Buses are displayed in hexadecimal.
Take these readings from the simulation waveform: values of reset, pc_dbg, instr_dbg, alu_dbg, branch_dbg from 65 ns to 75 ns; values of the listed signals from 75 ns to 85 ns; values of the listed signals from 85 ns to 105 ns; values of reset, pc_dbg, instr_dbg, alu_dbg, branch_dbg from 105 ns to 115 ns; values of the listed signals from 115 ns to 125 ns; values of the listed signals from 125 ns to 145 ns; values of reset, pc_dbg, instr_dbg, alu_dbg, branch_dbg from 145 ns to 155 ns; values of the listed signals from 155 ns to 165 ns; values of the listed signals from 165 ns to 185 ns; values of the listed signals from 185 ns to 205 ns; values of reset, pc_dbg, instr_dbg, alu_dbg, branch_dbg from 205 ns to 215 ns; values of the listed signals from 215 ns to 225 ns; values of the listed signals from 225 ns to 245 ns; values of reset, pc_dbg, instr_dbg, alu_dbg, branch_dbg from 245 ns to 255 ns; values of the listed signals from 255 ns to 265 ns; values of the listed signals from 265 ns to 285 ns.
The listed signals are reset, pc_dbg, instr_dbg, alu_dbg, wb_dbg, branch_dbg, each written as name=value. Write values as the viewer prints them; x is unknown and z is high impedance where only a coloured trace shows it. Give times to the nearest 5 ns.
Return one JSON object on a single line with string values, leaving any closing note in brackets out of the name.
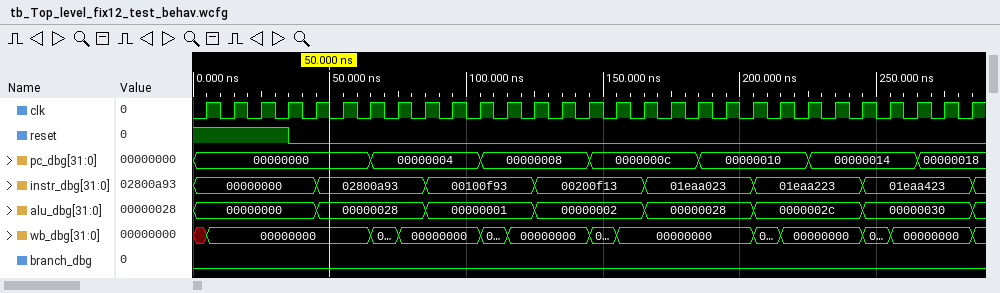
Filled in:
{"values of reset, pc_dbg, instr_dbg, alu_dbg, branch_dbg from 65 ns to 75 ns": "reset=0, pc_dbg=00000004, instr_dbg=02800a93, alu_dbg=00000028, branch_dbg=0", "values of the listed signals from 75 ns to 85 ns": "reset=0, pc_dbg=00000004, instr_dbg=02800a93, alu_dbg=00000028, wb_dbg=00000000, branch_dbg=0", "values of the listed signals from 85 ns to 105 ns": "reset=0, pc_dbg=00000004, instr_dbg=00100f93, alu_dbg=00000001, wb_dbg=00000000, branch_dbg=0", "values of reset, pc_dbg, instr_dbg, alu_dbg, branch_dbg from 105 ns to 115 ns": "reset=0, pc_dbg=00000008, instr_dbg=00100f93, alu_dbg=00000001, branch_dbg=0", "values of the listed signals from 115 ns to 125 ns": "reset=0, pc_dbg=00000008, instr_dbg=00100f93, alu_dbg=00000001, wb_dbg=00000000, branch_dbg=0", "values of the listed signals from 125 ns to 145 ns": "reset=0, pc_dbg=00000008, instr_dbg=00200f13, alu_dbg=00000002, wb_dbg=00000000, branch_dbg=0", "values of reset, pc_dbg, instr_dbg, alu_dbg, branch_dbg from 145 ns to 155 ns": "reset=0, pc_dbg=0000000c, instr_dbg=00200f13, alu_dbg=00000002, branch_dbg=0", "values of the listed signals from 155 ns to 165 ns": "reset=0, pc_dbg=0000000c, instr_dbg=00200f13, alu_dbg=00000002, wb_dbg=00000000, branch_dbg=0", "values of the listed signals from 165 ns to 185 ns": "reset=0, pc_dbg=0000000c, instr_dbg=01eaa023, alu_dbg=00000028, wb_dbg=00000000, branch_dbg=0", "values of the listed signals from 185 ns to 205 ns": "reset=0, pc_dbg=00000010, instr_dbg=01eaa023, alu_dbg=00000028, wb_dbg=00000000, branch_dbg=0", "values of reset, pc_dbg, instr_dbg, alu_dbg, branch_dbg from 205 ns to 215 ns": "reset=0, pc_dbg=00000010, instr_dbg=01eaa223, alu_dbg=0000002c, branch_dbg=0", "values of the listed signals from 215 ns to 225 ns": "reset=0, pc_dbg=00000010, instr_dbg=01eaa223, alu_dbg=0000002c, wb_dbg=00000000, branch_dbg=0", "values of the listed signals from 225 ns to 245 ns": "reset=0, pc_dbg=00000014, instr_dbg=01eaa223, alu_dbg=0000002c, wb_dbg=00000000, branch_dbg=0", "values of reset, pc_dbg, instr_dbg, alu_dbg, branch_dbg from 245 ns to 255 ns": "reset=0, pc_dbg=00000014, instr_dbg=01eaa423, alu_dbg=00000030, branch_dbg=0", "values of the listed signals from 255 ns to 265 ns": "reset=0, pc_dbg=00000014, instr_dbg=01eaa423, alu_dbg=00000030, wb_dbg=00000000, branch_dbg=0", "values of the listed signals from 265 ns to 285 ns": "reset=0, pc_dbg=00000018, instr_dbg=01eaa423, alu_dbg=00000030, wb_dbg=00000000, branch_dbg=0"}
